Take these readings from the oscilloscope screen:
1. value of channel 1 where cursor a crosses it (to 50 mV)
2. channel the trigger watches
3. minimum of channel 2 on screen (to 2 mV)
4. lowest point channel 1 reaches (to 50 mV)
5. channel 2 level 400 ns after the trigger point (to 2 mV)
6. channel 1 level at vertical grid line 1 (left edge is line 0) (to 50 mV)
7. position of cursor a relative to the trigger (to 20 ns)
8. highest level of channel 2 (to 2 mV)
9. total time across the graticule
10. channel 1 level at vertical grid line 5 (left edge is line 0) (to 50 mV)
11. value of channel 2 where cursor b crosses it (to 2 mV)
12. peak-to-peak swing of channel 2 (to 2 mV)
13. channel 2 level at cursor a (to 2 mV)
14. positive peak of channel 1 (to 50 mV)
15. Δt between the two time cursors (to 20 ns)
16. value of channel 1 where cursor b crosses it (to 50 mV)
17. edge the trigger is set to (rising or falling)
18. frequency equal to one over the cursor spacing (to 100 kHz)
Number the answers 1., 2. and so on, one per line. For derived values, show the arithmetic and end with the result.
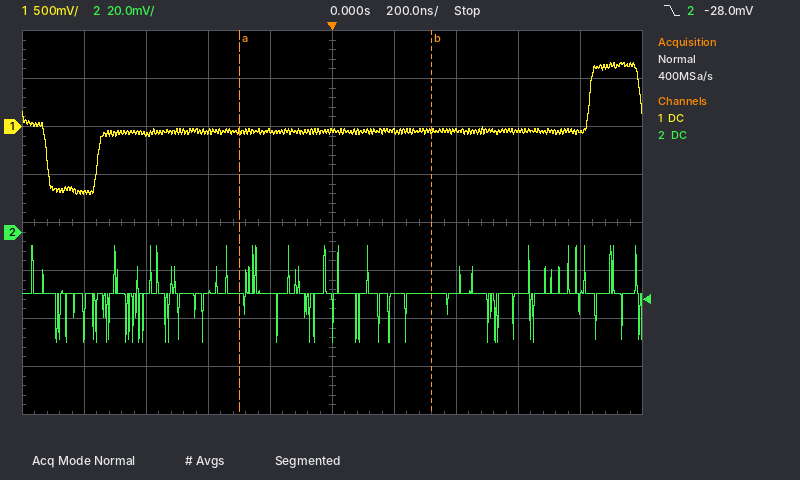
1. -50 mV
2. channel 2
3. -46 mV
4. -700 mV
5. -26 mV
6. -700 mV
7. -300 ns
8. -6 mV
9. 2 µs
10. -50 mV
11. -26 mV
12. -6 mV − (-46 mV) = 40 mV
13. -26 mV
14. 650 mV
15. 620 ns
16. -50 mV
17. falling
18. 1 / 620 ns ≈ 1.6 MHz
